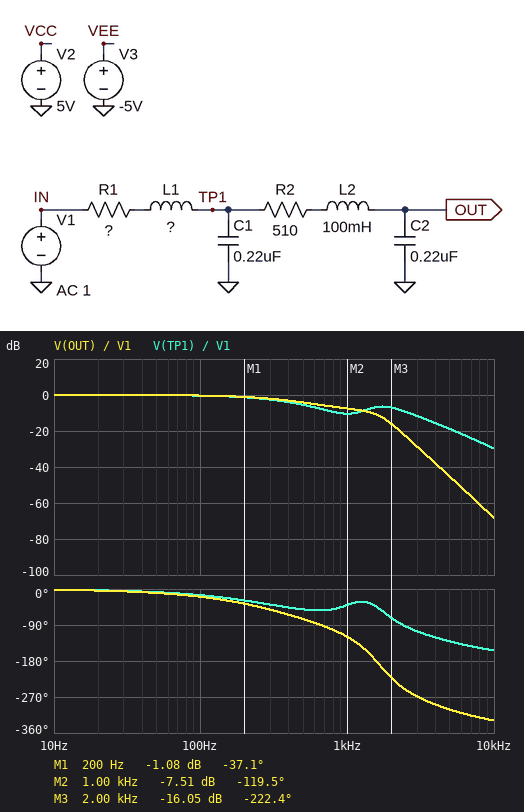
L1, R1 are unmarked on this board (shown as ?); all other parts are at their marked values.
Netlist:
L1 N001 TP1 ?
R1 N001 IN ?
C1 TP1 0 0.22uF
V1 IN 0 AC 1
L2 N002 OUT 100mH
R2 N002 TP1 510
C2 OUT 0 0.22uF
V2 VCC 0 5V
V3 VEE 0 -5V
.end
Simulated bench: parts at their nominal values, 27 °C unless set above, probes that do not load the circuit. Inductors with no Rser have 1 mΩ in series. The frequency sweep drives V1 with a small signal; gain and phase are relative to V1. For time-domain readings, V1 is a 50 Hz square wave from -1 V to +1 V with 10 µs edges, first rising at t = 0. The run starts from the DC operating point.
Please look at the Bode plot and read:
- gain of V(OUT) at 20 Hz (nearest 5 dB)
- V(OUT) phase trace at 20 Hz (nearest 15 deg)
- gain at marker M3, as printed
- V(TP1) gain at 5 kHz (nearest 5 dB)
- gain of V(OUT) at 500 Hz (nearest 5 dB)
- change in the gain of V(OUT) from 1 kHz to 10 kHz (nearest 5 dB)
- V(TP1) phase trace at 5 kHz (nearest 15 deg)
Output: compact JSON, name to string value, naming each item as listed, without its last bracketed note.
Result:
{"gain of V(OUT) at 20 Hz": "0 dB", "V(OUT) phase trace at 20 Hz": "0 deg", "gain at marker M3, as printed": "-16.05 dB", "V(TP1) gain at 5 kHz": "-20 dB", "gain of V(OUT) at 500 Hz": "-5 dB", "change in the gain of V(OUT) from 1 kHz to 10 kHz": "-60 dB", "V(TP1) phase trace at 5 kHz": "-135 deg"}
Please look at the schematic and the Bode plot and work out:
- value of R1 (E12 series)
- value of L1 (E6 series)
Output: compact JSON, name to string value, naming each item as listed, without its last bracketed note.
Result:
{"value of R1": "1 kΩ", "value of L1": "33 mH"}
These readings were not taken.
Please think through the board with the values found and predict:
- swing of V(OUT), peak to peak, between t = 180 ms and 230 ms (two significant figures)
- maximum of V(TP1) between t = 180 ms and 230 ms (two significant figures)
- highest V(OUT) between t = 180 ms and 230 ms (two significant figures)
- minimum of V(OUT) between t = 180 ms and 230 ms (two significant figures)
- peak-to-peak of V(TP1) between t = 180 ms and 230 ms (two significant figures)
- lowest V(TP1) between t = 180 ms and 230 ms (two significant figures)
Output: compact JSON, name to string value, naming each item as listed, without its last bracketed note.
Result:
{"swing of V(OUT), peak to peak, between t = 180 ms and 230 ms": "2.0 V", "maximum of V(TP1) between t = 180 ms and 230 ms": "1.0 V", "highest V(OUT) between t = 180 ms and 230 ms": "1.0 V", "minimum of V(OUT) between t = 180 ms and 230 ms": "-1.0 V", "peak-to-peak of V(TP1) between t = 180 ms and 230 ms": "2.0 V", "lowest V(TP1) between t = 180 ms and 230 ms": "-1.0 V"}
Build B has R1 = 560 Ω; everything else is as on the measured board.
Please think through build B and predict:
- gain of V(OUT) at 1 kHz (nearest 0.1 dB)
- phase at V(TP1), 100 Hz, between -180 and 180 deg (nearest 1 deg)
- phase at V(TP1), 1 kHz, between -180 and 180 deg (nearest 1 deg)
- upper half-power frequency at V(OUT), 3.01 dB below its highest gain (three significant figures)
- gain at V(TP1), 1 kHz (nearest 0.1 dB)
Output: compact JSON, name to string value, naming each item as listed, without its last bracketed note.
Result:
{"gain of V(OUT) at 1 kHz": "-3.9 dB", "phase at V(TP1), 100 Hz, between -180 and 180 deg": "-9 deg", "phase at V(TP1), 1 kHz, between -180 and 180 deg": "-39 deg", "upper half-power frequency at V(OUT), 3.01 dB below its highest gain": "853 Hz", "gain at V(TP1), 1 kHz": "-6.8 dB"}
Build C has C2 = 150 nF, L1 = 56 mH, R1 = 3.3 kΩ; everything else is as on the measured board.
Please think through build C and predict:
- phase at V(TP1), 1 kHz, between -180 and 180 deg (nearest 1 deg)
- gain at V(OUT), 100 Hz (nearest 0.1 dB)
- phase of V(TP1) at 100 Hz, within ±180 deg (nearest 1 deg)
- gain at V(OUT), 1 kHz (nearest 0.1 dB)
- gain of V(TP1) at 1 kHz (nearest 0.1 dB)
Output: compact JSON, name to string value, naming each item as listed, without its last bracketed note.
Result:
{"phase at V(TP1), 1 kHz, between -180 and 180 deg": "-64 deg", "gain at V(OUT), 100 Hz": "-2.0 dB", "phase of V(TP1) at 100 Hz, within ±180 deg": "-37 deg", "gain at V(OUT), 1 kHz": "-15.1 dB", "gain of V(TP1) at 1 kHz": "-19.1 dB"}
